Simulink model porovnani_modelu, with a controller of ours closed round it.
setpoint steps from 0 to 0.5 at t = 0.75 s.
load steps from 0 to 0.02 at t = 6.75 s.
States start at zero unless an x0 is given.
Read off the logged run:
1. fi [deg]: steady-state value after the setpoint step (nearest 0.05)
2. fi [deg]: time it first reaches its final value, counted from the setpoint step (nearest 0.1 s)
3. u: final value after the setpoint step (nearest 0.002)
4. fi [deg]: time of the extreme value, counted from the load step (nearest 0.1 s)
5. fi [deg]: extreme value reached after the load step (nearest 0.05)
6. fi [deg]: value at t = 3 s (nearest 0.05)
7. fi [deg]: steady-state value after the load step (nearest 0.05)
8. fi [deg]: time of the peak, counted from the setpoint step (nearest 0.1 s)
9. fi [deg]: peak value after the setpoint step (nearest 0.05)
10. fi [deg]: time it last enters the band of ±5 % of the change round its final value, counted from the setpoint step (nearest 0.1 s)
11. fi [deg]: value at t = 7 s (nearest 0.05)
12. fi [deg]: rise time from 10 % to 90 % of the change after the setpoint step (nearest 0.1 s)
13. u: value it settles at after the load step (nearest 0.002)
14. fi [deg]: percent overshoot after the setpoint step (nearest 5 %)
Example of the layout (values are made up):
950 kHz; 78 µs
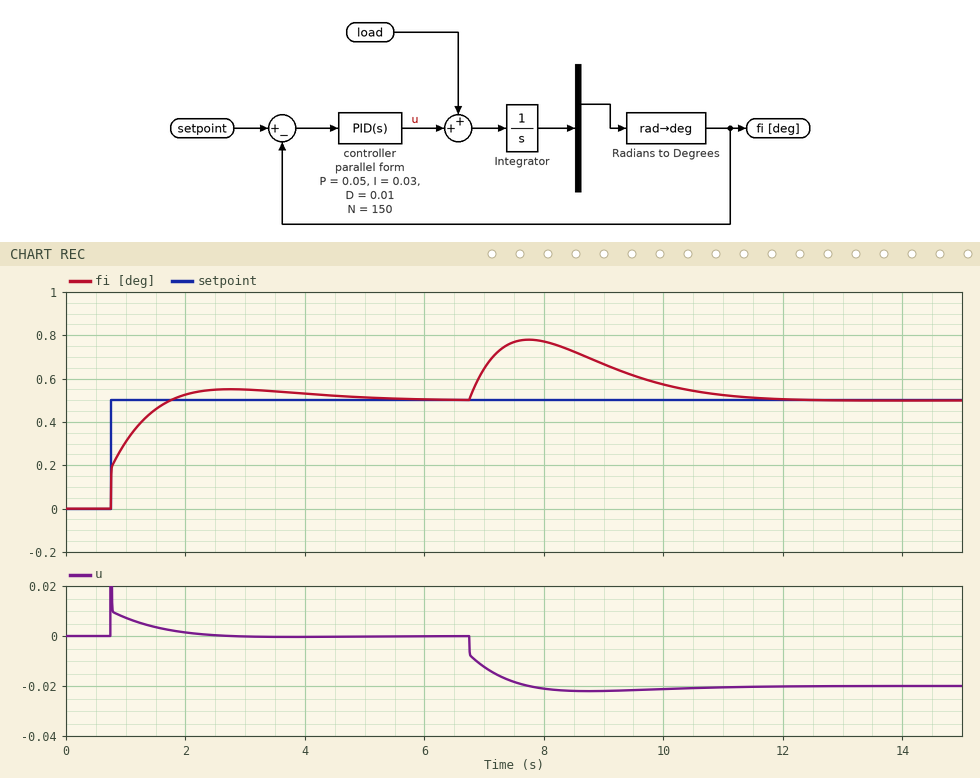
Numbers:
0.50; 1.0 s; 0.000; 1.0 s; 0.80; 0.55; 0.50; 2.0 s; 0.55; 3.5 s; 0.65; 0.7 s; -0.020; 10 %
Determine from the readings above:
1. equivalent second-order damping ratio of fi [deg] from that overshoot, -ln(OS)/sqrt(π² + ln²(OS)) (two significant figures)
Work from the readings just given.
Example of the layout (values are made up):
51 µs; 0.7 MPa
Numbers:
0.59
